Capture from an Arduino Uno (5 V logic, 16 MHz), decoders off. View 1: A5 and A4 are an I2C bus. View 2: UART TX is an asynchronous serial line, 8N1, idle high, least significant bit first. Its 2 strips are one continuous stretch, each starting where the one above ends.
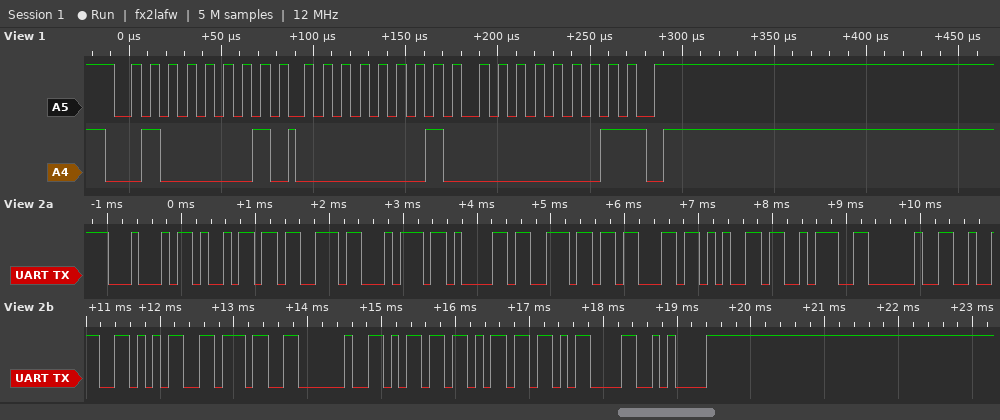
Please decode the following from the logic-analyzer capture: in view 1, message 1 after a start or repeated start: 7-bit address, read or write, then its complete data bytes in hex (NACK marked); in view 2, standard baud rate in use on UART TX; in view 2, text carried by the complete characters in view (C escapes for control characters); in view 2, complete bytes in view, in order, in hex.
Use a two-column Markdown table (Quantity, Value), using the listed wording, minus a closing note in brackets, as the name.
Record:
| Quantity | Value |
|---|---|
| in view 1, message 1 after a start or repeated start: 7-bit address, read or write, then its complete data bytes in hex | 0x20 read: 01 01 NACK |
| in view 2, standard baud rate in use on UART TX | 9600 baud |
| in view 2, text carried by the complete characters in view | "Distance: 257 mm\r\n" |
| in view 2, complete bytes in view, in order, in hex | 44 69 73 74 61 6E 63 65 3A 20 32 35 37 20 6D 6D 0D 0A |
